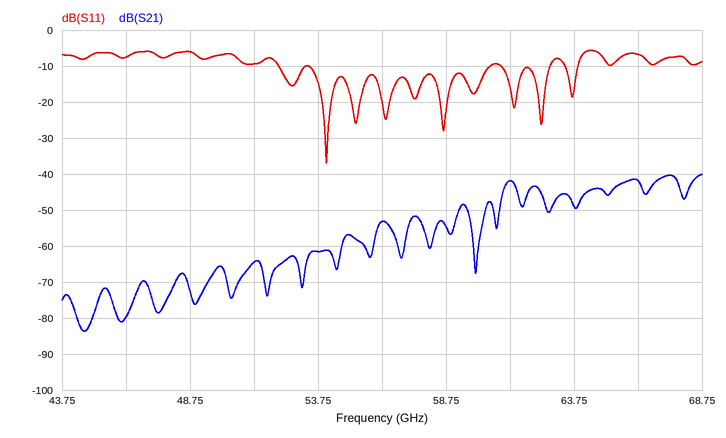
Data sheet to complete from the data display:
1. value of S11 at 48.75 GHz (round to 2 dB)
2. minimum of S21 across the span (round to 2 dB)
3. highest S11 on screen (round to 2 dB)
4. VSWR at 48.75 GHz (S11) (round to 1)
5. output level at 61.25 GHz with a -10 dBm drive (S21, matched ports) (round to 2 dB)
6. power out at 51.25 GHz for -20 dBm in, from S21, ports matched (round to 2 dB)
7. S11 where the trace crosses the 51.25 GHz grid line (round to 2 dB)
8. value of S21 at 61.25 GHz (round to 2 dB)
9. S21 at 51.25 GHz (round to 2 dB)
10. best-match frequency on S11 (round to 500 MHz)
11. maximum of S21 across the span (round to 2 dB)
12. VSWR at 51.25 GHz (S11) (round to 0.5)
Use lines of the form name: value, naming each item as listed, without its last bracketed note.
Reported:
value of S11 at 48.75 GHz: -6 dB
minimum of S21 across the span: -84 dB
highest S11 on screen: -6 dB
VSWR at 48.75 GHz (S11): 3
output level at 61.25 GHz with a -10 dBm drive (S21, matched ports): -52 dBm
power out at 51.25 GHz for -20 dBm in, from S21, ports matched: -84 dBm
S11 where the trace crosses the 51.25 GHz grid line: -10 dB
value of S21 at 61.25 GHz: -42 dB
S21 at 51.25 GHz: -64 dB
best-match frequency on S11: 54.0 GHz
maximum of S21 across the span: -40 dB
VSWR at 51.25 GHz (S11): 2.0
